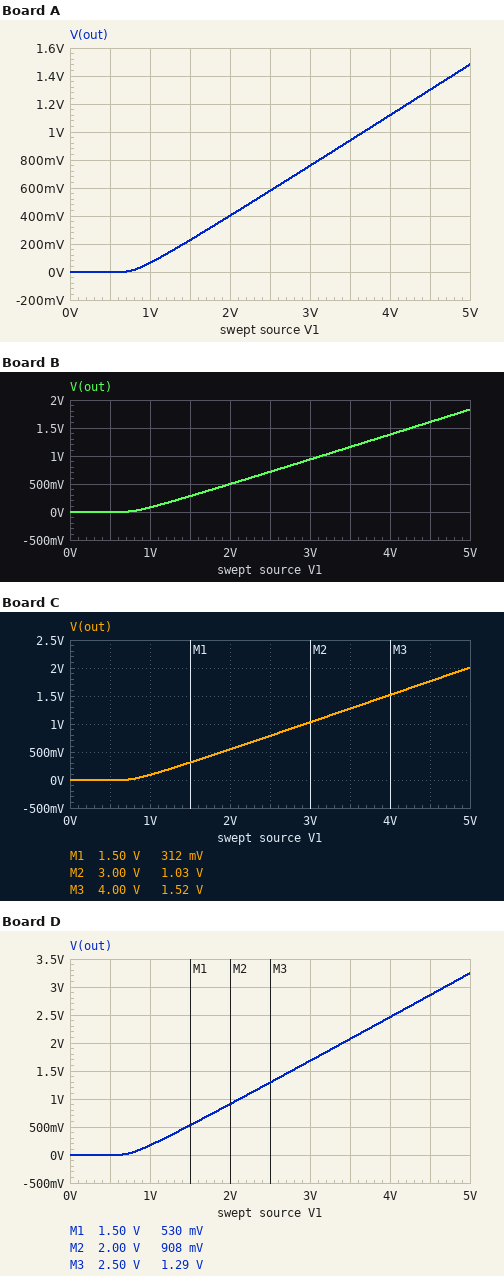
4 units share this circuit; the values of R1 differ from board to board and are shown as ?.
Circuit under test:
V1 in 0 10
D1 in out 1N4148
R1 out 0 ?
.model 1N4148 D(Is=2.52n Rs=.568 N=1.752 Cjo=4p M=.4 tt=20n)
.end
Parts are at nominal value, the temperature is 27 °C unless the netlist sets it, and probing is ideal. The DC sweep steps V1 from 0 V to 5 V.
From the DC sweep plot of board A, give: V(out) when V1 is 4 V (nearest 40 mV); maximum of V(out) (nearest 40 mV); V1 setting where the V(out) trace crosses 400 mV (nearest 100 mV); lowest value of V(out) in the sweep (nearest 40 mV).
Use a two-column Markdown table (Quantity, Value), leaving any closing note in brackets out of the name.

| Quantity | Value |
|---|---|
| V(out) when V1 is 4 V | 1.12 V |
| maximum of V(out) | 1.48 V |
| V1 setting where the V(out) trace crosses 400 mV | 2.0 V |
| lowest value of V(out) in the sweep | 0 V |
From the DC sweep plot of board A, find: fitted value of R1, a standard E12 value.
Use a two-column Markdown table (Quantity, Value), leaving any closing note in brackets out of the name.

| Quantity | Value |
|---|---|
| fitted value of R1, a standard E12 value | 0.33 Ω |
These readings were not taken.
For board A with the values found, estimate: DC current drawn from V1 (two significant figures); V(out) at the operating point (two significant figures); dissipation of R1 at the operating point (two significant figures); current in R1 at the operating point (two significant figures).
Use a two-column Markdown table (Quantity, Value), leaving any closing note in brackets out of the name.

| Quantity | Value |
|---|---|
| DC current drawn from V1 | 10 A |
| V(out) at the operating point | 3.3 V |
| dissipation of R1 at the operating point | 33 W |
| current in R1 at the operating point | 10 A |
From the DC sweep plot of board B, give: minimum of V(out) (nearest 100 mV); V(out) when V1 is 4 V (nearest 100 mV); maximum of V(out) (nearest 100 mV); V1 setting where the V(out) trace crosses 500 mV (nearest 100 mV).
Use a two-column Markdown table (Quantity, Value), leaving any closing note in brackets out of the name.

| Quantity | Value |
|---|---|
| minimum of V(out) | 0 V |
| V(out) when V1 is 4 V | 1.4 V |
| maximum of V(out) | 1.8 V |
| V1 setting where the V(out) trace crosses 500 mV | 2.0 V |
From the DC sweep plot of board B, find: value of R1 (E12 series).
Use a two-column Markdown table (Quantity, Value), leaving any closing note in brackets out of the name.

| Quantity | Value |
|---|---|
| value of R1 | 0.47 Ω |
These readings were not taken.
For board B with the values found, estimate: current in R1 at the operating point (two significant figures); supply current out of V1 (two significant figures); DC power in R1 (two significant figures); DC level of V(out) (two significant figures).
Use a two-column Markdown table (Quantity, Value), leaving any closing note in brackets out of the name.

| Quantity | Value |
|---|---|
| current in R1 at the operating point | 8.7 A |
| supply current out of V1 | 8.7 A |
| DC power in R1 | 35 W |
| DC level of V(out) | 4.1 V |
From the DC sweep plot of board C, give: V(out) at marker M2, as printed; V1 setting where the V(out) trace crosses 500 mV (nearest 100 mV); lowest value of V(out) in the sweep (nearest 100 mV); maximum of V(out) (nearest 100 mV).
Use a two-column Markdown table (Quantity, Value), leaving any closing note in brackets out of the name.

| Quantity | Value |
|---|---|
| V(out) at marker M2, as printed | 1.03 V |
| V1 setting where the V(out) trace crosses 500 mV | 1.9 V |
| lowest value of V(out) in the sweep | 0 V |
| maximum of V(out) | 2.0 V |
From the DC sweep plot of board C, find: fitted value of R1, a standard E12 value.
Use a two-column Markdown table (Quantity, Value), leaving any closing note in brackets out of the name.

| Quantity | Value |
|---|---|
| fitted value of R1, a standard E12 value | 0.56 Ω |
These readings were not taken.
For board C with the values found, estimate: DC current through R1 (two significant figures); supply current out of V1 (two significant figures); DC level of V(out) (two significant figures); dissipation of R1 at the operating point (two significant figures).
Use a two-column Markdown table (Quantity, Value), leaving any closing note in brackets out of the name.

| Quantity | Value |
|---|---|
| DC current through R1 | 8.0 A |
| supply current out of V1 | 8.0 A |
| DC level of V(out) | 4.5 V |
| dissipation of R1 at the operating point | 36 W |
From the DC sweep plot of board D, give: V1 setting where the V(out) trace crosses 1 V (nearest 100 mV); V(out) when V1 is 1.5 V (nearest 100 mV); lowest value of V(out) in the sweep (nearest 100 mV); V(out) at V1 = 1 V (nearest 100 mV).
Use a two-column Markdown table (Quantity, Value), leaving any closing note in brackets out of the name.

| Quantity | Value |
|---|---|
| V1 setting where the V(out) trace crosses 1 V | 2.1 V |
| V(out) when V1 is 1.5 V | 500 mV |
| lowest value of V(out) in the sweep | 0 V |
| V(out) at V1 = 1 V | 200 mV |
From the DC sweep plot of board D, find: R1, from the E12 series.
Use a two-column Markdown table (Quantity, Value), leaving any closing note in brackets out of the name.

| Quantity | Value |
|---|---|
| R1, from the E12 series | 2.2 Ω |
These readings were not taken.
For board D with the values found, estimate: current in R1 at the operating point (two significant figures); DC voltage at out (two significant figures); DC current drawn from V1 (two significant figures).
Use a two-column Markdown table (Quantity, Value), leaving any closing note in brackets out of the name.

| Quantity | Value |
|---|---|
| current in R1 at the operating point | 3.3 A |
| DC voltage at out | 7.2 V |
| DC current drawn from V1 | 3.3 A |
